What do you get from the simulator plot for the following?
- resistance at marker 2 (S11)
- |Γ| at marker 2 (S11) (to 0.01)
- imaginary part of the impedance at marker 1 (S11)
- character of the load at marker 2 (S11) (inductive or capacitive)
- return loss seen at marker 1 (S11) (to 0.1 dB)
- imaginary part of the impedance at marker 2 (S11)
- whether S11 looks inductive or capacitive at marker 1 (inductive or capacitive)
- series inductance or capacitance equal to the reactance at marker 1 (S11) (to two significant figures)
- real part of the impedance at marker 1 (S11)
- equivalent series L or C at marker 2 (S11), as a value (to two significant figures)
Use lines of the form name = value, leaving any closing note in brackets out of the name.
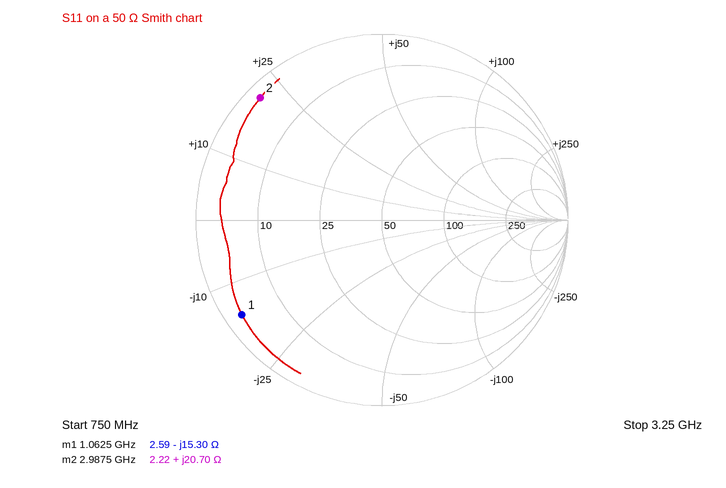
resistance at marker 2 = 2.22 Ω
|Γ| at marker 2 (S11) = 0.93
imaginary part of the impedance at marker 1 = -15.30 Ω
character of the load at marker 2 (S11) = inductive
return loss seen at marker 1 (S11) = 0.8 dB
imaginary part of the impedance at marker 2 = +20.70 Ω
whether S11 looks inductive or capacitive at marker 1 = capacitive
series inductance or capacitance equal to the reactance at marker 1 (S11) = 9.8 pF
real part of the impedance at marker 1 = 2.59 Ω
equivalent series L or C at marker 2 (S11), as a value = 1.1 nH
